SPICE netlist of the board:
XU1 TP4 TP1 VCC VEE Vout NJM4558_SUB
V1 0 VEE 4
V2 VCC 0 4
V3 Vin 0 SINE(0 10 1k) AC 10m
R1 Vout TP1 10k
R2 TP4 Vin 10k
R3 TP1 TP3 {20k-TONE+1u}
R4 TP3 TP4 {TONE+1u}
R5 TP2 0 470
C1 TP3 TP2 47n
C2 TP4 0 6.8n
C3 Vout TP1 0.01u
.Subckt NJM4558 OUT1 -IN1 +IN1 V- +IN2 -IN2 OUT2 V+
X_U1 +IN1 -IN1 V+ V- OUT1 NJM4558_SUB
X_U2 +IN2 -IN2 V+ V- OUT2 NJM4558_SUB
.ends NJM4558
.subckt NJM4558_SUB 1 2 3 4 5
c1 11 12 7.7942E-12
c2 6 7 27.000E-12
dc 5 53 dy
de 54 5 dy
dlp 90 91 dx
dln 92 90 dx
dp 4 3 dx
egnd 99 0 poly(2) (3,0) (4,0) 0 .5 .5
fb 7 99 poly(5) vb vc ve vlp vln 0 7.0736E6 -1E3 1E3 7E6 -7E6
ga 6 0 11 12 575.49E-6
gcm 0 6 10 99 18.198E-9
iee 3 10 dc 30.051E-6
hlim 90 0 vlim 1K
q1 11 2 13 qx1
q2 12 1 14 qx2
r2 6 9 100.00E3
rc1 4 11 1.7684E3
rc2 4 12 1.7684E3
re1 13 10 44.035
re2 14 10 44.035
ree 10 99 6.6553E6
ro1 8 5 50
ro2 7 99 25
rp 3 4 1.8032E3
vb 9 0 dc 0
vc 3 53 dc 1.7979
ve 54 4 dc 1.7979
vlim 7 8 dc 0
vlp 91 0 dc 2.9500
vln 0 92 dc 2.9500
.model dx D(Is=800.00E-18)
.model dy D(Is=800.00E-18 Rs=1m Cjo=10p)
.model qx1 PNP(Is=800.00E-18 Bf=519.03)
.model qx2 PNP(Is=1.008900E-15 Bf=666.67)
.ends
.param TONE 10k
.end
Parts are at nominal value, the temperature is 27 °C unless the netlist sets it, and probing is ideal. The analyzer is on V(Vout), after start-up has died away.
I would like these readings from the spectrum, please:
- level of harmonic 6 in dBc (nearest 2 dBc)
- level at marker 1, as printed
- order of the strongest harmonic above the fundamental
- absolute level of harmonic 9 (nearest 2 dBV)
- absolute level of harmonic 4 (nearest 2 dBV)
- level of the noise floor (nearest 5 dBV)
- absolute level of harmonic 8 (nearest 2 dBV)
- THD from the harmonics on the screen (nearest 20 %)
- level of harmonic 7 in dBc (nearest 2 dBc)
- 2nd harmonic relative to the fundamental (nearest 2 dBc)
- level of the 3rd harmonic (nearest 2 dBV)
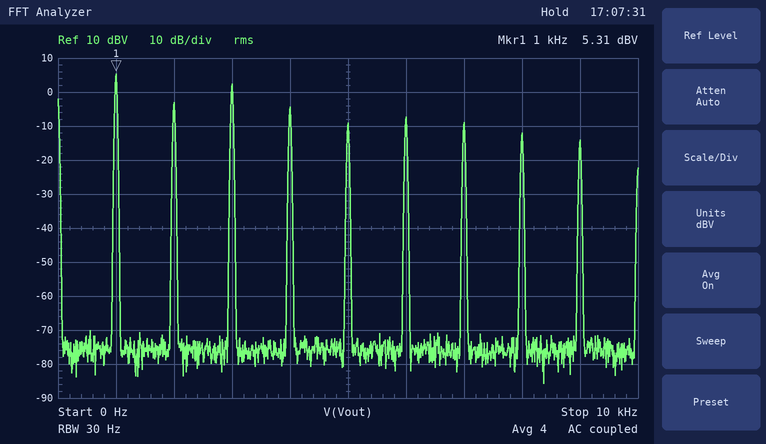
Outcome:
-12 dBc
5.31 dBV
3
-14 dBV
-4 dBV
-75 dBV
-12 dBV
100 %
-14 dBc
-8 dBc
2 dBV
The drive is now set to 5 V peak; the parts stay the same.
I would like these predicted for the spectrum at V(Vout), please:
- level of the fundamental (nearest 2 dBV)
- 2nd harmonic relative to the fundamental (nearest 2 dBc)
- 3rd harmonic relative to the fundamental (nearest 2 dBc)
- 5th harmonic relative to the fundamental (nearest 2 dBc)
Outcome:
8 dBV
-54 dBc
-18 dBc
-32 dBc
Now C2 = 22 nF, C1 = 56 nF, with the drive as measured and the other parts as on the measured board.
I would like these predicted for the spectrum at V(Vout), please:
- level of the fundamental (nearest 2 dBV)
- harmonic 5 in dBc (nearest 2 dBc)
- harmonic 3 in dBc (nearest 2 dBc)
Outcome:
8 dBV
-26 dBc
-12 dBc
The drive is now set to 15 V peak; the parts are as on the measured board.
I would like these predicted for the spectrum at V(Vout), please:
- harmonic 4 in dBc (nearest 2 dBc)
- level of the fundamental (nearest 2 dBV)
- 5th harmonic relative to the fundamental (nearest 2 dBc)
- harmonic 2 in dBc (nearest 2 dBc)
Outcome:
-18 dBc
-2 dBV
-2 dBc
4 dBc
